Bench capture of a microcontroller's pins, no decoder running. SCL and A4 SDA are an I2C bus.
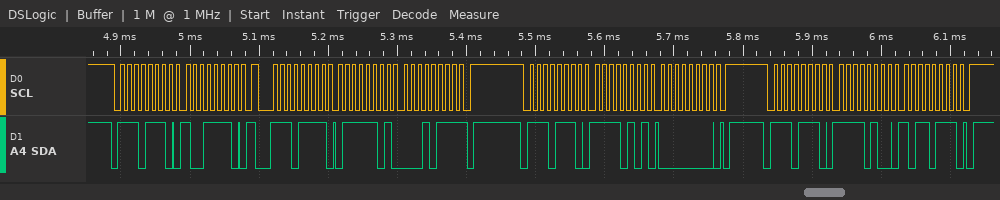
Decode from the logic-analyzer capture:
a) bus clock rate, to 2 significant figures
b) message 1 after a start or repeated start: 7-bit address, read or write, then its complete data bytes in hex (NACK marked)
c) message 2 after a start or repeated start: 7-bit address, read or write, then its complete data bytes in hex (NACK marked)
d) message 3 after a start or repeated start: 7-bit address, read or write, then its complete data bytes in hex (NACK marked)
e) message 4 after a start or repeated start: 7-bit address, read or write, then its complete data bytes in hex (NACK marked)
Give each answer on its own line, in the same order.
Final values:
100 kHz
0x77 write: 9E
0x77 read: 7D 17 NACK
0x77 write: F5 00
0x77 write: F4 B7
